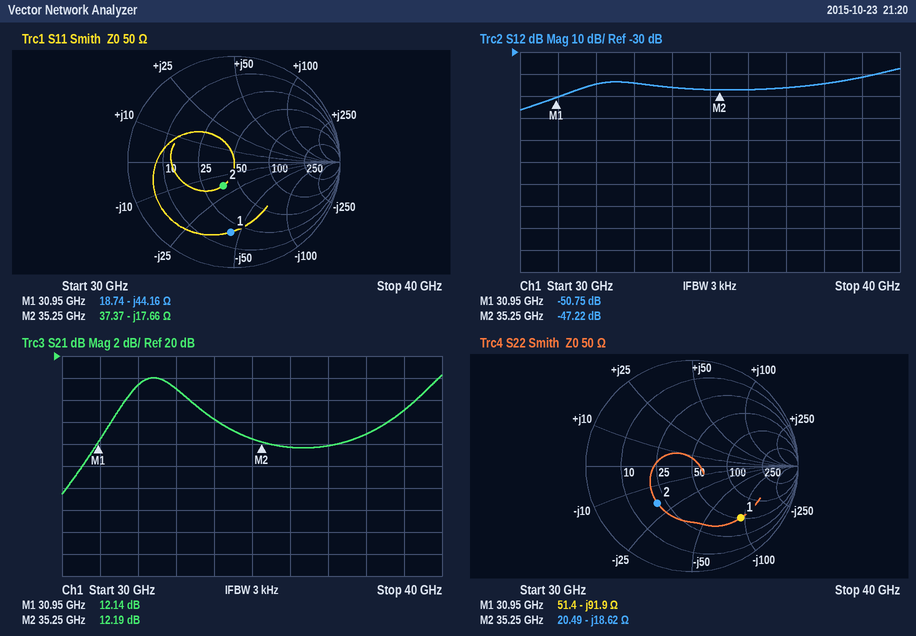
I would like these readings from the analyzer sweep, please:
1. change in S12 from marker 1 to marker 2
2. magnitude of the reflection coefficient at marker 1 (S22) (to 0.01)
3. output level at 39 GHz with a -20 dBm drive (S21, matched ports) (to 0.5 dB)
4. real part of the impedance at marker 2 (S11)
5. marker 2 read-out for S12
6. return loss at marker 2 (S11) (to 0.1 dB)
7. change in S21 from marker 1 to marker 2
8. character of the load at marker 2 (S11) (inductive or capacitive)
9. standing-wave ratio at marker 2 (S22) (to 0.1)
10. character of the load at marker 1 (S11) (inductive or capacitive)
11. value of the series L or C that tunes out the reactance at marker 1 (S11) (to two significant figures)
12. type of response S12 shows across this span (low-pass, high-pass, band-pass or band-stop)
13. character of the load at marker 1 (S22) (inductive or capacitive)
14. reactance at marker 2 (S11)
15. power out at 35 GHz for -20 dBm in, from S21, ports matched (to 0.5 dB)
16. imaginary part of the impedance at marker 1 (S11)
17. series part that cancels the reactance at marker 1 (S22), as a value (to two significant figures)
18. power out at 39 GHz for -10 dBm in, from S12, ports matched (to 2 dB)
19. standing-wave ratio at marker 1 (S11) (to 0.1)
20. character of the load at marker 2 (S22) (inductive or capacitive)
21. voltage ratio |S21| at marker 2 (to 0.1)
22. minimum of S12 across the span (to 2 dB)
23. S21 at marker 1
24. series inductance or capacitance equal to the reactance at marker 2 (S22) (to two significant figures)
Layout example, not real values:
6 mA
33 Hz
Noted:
3.53 dB
0.67
-5.0 dBm
37.37 Ω
-47.22 dB
12.3 dB
0.05 dB
capacitive
2.8
capacitive
230 pH
high-pass
capacitive
-17.66 Ω
-7.5 dBm
-44.16 Ω
470 pH
-52 dBm
4.9
capacitive
4.1
-56 dB
12.14 dB
240 fF
